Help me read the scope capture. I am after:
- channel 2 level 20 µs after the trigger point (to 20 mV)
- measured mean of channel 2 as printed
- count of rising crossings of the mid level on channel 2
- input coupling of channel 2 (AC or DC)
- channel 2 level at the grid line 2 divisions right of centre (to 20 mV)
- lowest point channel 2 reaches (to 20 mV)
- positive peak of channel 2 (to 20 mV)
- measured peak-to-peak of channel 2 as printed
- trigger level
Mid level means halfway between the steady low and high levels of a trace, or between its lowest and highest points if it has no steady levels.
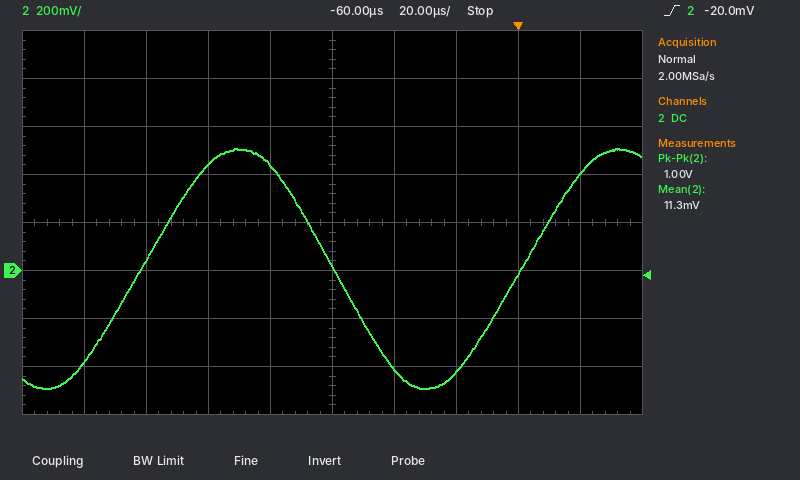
400 mV
11.3 mV
2
DC
-420 mV
-500 mV
500 mV
1.00 V
-20.0 mV
